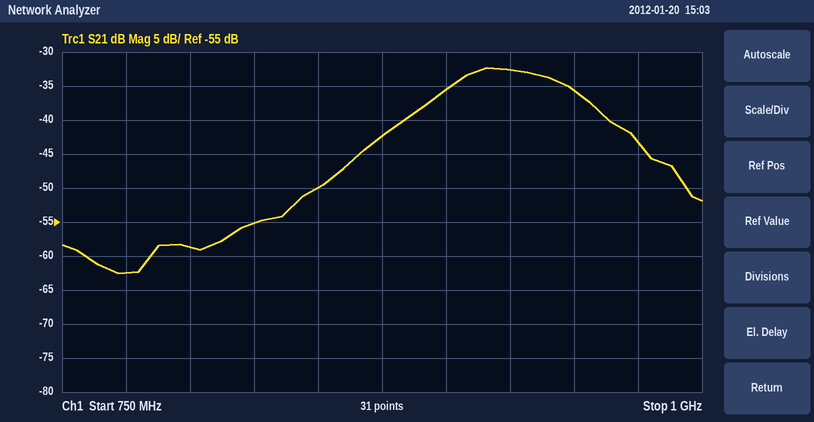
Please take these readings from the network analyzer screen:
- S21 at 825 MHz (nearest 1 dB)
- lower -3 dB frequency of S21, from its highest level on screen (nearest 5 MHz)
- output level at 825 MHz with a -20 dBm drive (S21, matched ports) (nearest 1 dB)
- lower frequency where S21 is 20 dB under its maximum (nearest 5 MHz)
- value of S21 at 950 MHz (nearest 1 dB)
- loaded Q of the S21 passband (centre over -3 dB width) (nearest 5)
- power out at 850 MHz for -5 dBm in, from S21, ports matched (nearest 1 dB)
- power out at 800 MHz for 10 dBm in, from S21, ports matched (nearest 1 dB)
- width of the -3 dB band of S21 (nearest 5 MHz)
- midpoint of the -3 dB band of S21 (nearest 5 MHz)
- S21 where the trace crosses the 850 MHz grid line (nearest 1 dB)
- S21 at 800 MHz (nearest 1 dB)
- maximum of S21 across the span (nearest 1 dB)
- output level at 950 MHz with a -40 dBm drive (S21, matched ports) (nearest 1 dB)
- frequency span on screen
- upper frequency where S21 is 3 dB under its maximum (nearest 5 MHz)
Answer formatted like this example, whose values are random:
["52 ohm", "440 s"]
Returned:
["-55 dB", "900 MHz", "-75 dBm", "840 MHz", "-36 dB", "20", "-55 dBm", "-49 dBm", "50 MHz", "925 MHz", "-50 dB", "-59 dB", "-32 dB", "-76 dBm", "250 MHz", "950 MHz"]
